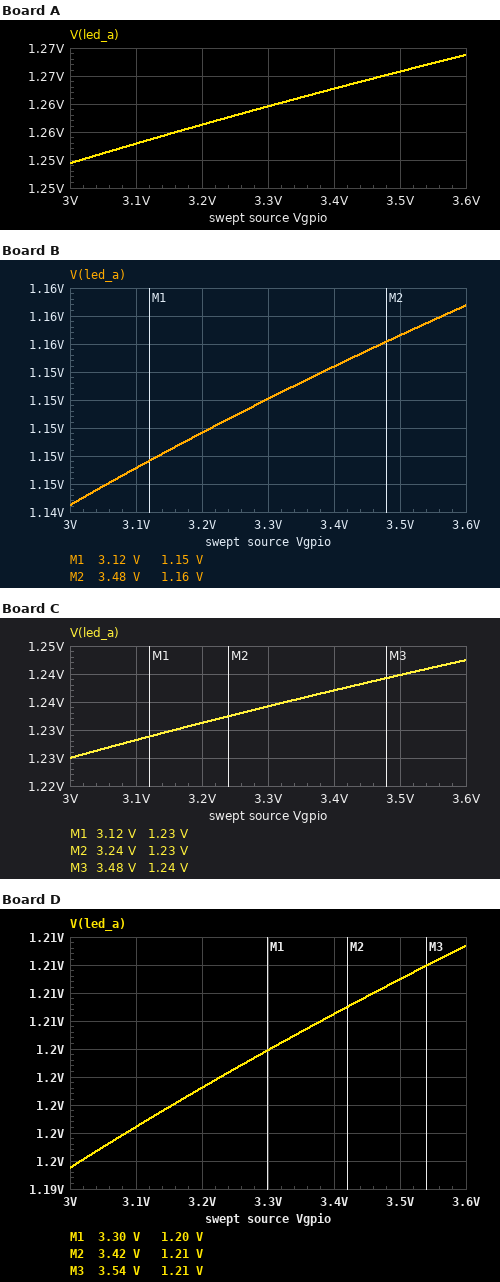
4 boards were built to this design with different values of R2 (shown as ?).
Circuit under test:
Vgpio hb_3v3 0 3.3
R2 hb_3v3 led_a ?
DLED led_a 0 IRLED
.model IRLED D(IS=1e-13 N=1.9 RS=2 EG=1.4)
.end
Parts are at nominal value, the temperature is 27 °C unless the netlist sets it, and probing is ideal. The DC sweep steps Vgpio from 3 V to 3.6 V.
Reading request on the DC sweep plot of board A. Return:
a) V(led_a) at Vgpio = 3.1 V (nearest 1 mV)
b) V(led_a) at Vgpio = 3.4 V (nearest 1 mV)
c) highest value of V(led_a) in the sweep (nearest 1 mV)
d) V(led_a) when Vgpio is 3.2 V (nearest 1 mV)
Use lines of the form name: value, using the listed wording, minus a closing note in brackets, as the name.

V(led_a) at Vgpio = 3.1 V: 1.253 V
V(led_a) at Vgpio = 3.4 V: 1.263 V
highest value of V(led_a) in the sweep: 1.269 V
V(led_a) when Vgpio is 3.2 V: 1.256 V
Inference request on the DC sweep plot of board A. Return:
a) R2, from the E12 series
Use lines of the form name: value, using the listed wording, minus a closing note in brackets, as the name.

R2, from the E12 series: 220 Ω
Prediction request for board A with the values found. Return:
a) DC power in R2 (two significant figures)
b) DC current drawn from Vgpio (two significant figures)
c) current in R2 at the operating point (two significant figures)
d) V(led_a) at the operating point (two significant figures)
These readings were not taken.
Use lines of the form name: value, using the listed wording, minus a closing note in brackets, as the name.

DC power in R2: 19 mW
DC current drawn from Vgpio: 9.3 mA
current in R2 at the operating point: 9.3 mA
V(led_a) at the operating point: 1.3 V
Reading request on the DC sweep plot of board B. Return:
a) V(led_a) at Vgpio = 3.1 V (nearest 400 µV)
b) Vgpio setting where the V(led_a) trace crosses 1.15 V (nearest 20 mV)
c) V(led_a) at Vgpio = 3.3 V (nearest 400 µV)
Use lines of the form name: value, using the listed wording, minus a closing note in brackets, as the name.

V(led_a) at Vgpio = 3.1 V: 1.1472 V
Vgpio setting where the V(led_a) trace crosses 1.15 V: 3.30 V
V(led_a) at Vgpio = 3.3 V: 1.1520 V
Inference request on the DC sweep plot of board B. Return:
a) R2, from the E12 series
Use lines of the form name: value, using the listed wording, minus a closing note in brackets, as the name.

R2, from the E12 series: 1.5 kΩ
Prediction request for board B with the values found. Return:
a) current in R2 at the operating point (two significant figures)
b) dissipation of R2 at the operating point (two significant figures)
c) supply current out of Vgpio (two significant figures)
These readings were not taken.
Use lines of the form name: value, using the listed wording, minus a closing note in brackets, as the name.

current in R2 at the operating point: 1.4 mA
dissipation of R2 at the operating point: 3.1 mW
supply current out of Vgpio: 1.4 mA
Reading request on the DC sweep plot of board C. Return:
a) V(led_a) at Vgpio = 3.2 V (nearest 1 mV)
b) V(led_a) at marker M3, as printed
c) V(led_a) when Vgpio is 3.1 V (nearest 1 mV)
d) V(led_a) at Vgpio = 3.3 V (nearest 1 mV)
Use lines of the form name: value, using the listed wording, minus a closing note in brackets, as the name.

V(led_a) at Vgpio = 3.2 V: 1.231 V
V(led_a) at marker M3, as printed: 1.24 V
V(led_a) when Vgpio is 3.1 V: 1.228 V
V(led_a) at Vgpio = 3.3 V: 1.234 V
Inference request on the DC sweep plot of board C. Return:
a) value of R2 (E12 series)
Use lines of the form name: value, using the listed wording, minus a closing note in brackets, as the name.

value of R2: 330 Ω
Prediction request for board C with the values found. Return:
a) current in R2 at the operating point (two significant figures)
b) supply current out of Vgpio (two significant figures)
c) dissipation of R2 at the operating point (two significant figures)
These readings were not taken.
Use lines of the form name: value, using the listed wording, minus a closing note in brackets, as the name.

current in R2 at the operating point: 6.3 mA
supply current out of Vgpio: 6.3 mA
dissipation of R2 at the operating point: 13 mW
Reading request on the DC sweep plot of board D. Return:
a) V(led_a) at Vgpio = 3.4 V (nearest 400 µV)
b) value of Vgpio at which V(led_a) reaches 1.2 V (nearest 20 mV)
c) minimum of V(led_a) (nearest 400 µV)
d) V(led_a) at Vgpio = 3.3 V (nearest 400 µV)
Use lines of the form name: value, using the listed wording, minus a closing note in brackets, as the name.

V(led_a) at Vgpio = 3.4 V: 1.2064 V
value of Vgpio at which V(led_a) reaches 1.2 V: 3.08 V
minimum of V(led_a): 1.1956 V
V(led_a) at Vgpio = 3.3 V: 1.2040 V
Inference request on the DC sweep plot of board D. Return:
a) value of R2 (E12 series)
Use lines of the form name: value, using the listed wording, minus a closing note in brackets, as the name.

value of R2: 560 Ω
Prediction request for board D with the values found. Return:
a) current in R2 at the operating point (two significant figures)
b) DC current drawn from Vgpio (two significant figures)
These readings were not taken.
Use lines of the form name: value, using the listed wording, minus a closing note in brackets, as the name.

current in R2 at the operating point: 3.7 mA
DC current drawn from Vgpio: 3.7 mA
